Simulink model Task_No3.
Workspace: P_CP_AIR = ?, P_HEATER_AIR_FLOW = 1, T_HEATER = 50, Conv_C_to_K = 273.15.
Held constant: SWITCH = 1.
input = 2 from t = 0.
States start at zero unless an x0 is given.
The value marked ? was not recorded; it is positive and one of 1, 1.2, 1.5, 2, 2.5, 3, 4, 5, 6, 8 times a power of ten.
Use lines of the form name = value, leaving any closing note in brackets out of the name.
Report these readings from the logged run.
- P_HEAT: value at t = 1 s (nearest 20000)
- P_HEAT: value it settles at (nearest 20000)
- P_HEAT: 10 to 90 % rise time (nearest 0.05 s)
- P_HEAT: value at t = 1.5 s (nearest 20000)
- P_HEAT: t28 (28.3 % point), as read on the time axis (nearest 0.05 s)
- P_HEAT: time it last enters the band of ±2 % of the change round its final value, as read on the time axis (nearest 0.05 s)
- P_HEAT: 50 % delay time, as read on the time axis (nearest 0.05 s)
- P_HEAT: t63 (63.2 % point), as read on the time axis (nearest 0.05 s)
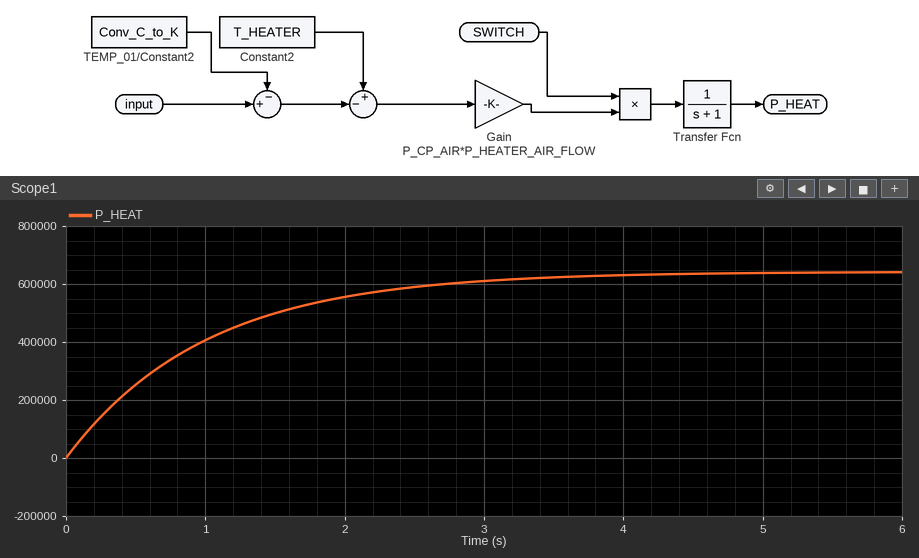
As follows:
P_HEAT: value at t = 1 s = 400000
P_HEAT: value it settles at = 640000
P_HEAT: 10 to 90 % rise time = 2.20 s
P_HEAT: value at t = 1.5 s = 500000
P_HEAT: t28 (28.3 % point), as read on the time axis = 0.35 s
P_HEAT: time it last enters the band of ±2 % of the change round its final value, as read on the time axis = 3.90 s
P_HEAT: 50 % delay time, as read on the time axis = 0.70 s
P_HEAT: t63 (63.2 % point), as read on the time axis = 1.00 s
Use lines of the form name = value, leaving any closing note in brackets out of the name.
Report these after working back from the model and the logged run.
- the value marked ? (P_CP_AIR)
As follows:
the value marked ? = 2000
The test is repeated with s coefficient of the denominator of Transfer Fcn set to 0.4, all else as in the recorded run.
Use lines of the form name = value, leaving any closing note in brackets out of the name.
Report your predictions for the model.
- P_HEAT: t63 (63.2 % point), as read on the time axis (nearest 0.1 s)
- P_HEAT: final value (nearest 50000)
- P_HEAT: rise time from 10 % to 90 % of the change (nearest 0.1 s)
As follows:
P_HEAT: t63 (63.2 % point), as read on the time axis = 0.4 s
P_HEAT: final value = 650000
P_HEAT: rise time from 10 % to 90 % of the change = 0.9 s
